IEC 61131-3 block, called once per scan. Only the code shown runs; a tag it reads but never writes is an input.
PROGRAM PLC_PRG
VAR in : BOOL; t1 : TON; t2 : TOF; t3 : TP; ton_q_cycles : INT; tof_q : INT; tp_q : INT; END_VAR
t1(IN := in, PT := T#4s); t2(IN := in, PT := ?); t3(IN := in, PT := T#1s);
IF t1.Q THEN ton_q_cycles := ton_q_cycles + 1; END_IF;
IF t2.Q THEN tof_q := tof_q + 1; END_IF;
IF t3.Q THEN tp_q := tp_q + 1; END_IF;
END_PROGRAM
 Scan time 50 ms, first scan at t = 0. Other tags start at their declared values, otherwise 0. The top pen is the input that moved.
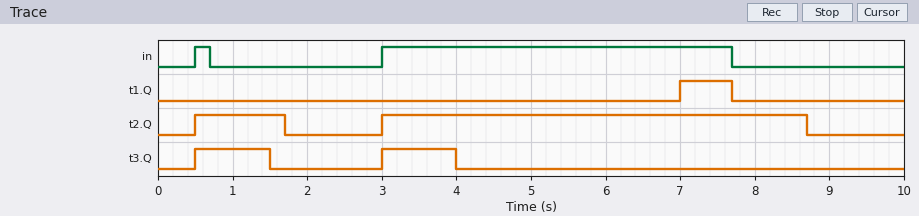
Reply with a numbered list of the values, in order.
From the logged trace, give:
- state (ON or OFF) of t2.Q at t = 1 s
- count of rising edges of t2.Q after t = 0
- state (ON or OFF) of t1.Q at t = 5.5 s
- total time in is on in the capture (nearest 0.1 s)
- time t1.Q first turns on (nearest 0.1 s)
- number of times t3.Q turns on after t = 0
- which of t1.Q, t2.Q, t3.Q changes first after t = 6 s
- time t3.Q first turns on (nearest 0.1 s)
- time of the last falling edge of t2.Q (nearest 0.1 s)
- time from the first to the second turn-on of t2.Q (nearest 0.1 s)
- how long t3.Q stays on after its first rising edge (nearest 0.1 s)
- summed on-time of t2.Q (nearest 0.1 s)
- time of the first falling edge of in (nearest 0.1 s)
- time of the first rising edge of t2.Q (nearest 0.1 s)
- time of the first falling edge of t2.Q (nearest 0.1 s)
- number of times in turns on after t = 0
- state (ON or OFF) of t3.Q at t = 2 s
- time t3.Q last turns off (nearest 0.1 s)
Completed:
1. ON
2. 2
3. OFF
4. 4.9 s
5. 7.0 s
6. 2
7. t1.Q
8. 0.5 s
9. 8.7 s
10. 2.5 s
11. 1.0 s
12. 6.9 s
13. 0.7 s
14. 0.5 s
15. 1.7 s
16. 2
17. OFF
18. 4.0 s
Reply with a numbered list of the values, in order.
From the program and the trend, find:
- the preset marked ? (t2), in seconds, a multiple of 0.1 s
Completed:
1. 1.0 s
